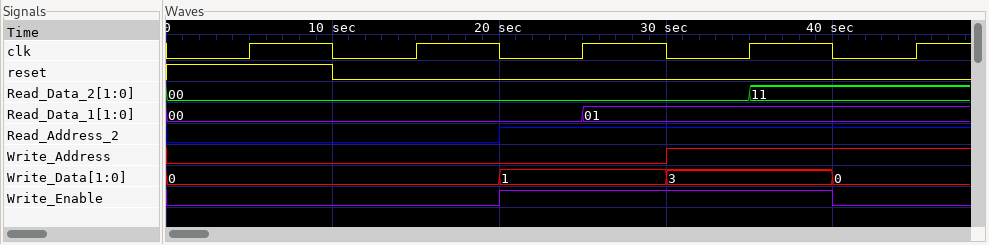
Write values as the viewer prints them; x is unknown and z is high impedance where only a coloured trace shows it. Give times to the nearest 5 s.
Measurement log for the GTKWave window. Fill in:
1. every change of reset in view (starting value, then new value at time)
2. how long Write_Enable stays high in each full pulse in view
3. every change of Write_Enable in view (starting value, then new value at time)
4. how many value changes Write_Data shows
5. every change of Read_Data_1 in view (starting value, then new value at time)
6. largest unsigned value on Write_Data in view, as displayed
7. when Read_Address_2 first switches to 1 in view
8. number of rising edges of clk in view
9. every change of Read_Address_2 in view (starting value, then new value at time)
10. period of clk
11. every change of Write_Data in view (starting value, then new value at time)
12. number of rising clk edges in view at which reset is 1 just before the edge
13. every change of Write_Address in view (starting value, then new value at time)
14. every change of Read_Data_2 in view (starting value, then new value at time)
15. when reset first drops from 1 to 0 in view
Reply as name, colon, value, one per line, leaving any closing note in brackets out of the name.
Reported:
every change of reset in view: 1, 0 at 10 s
how long Write_Enable stays high in each full pulse in view: 20 s
every change of Write_Enable in view: 0, 1 at 20 s, 0 at 40 s
how many value changes Write_Data shows: 3
every change of Read_Data_1 in view: 00, 01 at 25 s
largest unsigned value on Write_Data in view, as displayed: 3
when Read_Address_2 first switches to 1 in view: 20 s
number of rising edges of clk in view: 5
every change of Read_Address_2 in view: 0, 1 at 20 s
period of clk: 10 s
every change of Write_Data in view: 0, 1 at 20 s, 3 at 30 s, 0 at 40 s
number of rising clk edges in view at which reset is 1 just before the edge: 1
every change of Write_Address in view: 0, 1 at 30 s
every change of Read_Data_2 in view: 00, 11 at 35 s
when reset first drops from 1 to 0 in view: 10 s
